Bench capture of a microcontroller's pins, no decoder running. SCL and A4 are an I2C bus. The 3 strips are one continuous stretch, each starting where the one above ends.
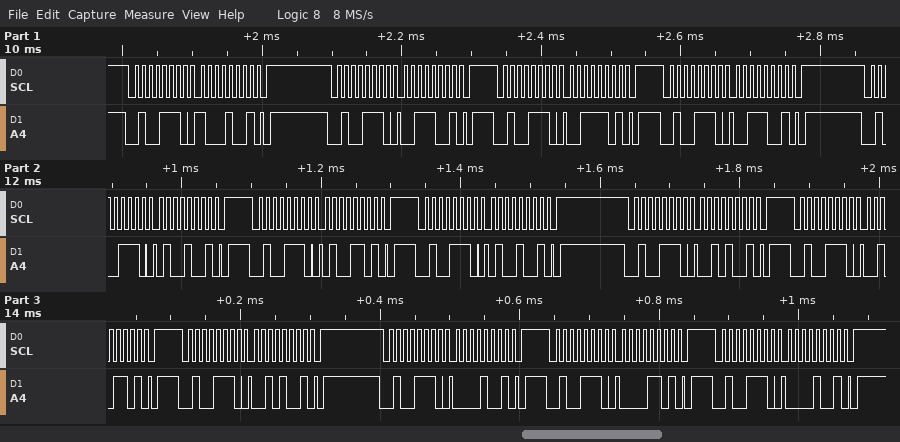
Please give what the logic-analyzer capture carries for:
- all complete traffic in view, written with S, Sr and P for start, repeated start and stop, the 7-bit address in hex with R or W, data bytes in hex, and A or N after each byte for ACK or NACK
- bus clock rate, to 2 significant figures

S 27W A 89 A P S 27W A 39 A P S 27W A 3D A P S 27W A 39 A P S 27W A 49 A P S 27W A 4D A P S 27W A 49 A P S 27W A 29 A P S 27W A 2D A P S 27W A 29 A P S 27W A 09 A P S 27W A 0D A P S 27W A 09 A P
100 kHz
